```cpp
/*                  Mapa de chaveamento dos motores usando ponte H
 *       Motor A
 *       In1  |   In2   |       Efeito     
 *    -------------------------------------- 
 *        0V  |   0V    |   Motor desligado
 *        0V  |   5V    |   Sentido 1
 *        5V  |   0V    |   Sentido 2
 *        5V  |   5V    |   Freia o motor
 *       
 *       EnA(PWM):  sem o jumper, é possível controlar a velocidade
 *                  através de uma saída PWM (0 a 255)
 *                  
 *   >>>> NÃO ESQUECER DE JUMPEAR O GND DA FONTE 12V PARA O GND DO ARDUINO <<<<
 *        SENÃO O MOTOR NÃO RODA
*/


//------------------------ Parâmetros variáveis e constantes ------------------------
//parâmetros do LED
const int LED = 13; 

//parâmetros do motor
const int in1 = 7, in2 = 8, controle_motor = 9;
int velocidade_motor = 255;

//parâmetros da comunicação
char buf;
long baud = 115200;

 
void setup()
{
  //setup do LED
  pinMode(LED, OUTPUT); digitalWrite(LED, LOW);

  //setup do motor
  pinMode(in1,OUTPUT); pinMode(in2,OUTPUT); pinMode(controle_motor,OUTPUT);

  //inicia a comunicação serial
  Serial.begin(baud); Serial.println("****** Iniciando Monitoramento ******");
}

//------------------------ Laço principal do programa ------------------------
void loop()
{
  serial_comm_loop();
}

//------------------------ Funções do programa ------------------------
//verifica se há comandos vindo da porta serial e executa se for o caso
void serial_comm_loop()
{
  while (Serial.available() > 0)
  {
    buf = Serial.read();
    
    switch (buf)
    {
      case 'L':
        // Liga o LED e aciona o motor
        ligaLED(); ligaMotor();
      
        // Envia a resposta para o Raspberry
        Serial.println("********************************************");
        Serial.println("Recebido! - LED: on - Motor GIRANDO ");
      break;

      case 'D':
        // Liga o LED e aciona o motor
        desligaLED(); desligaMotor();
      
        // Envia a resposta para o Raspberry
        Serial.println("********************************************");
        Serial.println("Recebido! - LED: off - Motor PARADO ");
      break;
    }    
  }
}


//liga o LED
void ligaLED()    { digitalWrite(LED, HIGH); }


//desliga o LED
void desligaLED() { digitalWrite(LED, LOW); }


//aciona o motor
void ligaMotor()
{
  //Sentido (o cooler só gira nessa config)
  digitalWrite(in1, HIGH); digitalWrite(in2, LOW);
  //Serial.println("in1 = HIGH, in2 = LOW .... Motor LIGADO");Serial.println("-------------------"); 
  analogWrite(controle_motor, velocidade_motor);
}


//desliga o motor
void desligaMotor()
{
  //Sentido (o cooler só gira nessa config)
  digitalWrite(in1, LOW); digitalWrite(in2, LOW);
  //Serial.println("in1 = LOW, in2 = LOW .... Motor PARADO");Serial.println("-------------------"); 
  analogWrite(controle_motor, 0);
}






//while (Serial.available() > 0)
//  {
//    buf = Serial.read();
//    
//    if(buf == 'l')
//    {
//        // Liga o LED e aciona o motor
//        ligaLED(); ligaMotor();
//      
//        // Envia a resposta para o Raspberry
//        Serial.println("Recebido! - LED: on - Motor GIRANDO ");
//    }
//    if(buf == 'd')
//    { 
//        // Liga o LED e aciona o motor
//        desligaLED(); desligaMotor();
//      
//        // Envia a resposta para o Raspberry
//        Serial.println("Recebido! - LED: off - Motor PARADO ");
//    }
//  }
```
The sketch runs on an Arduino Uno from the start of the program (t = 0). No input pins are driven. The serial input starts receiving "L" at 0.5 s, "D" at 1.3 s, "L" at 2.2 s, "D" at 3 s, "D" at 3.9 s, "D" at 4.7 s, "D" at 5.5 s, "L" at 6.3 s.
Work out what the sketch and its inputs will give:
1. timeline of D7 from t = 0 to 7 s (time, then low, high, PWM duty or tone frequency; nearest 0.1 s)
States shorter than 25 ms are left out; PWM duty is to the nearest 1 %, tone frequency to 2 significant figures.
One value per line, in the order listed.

0 s low; 0.5 s high; 1.3 s low; 2.2 s high; 3 s low; 6.3 s high
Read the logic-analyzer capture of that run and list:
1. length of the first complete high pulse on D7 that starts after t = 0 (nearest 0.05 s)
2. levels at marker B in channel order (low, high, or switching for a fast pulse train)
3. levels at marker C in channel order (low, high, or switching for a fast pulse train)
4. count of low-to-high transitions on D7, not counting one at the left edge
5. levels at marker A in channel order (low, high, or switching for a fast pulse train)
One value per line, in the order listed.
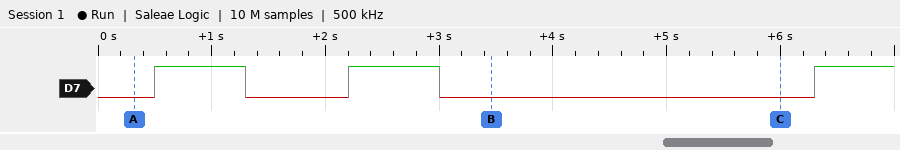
0.80 s
D7 low
D7 low
3
D7 low
